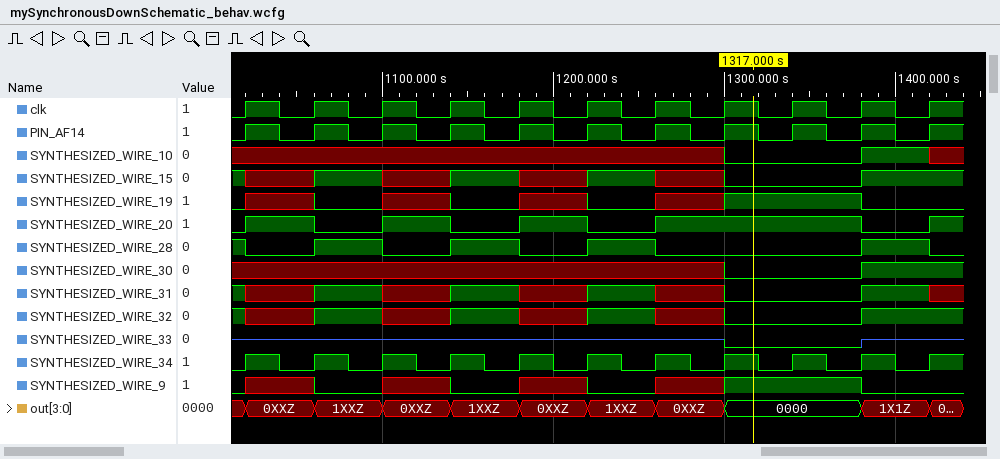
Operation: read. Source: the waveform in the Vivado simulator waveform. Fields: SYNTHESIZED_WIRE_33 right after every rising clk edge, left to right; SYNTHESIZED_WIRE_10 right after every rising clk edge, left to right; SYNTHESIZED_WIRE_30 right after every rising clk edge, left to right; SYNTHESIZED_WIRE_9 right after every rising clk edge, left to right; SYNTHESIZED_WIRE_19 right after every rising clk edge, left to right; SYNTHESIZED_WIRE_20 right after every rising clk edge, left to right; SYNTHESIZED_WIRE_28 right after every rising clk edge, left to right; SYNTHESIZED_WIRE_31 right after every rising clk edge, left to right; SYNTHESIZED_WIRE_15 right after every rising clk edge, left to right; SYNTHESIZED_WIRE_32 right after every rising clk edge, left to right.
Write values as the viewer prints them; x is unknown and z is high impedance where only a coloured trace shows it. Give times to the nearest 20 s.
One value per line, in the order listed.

z z z z z z z 0 0 z z
x x x x x x x 0 0 1 x
x x x x x x x 0 0 1 1
x 0 x 0 x 0 x 1 1 0 0
x 0 x 0 x 0 x 1 1 0 0
1 0 1 0 1 0 1 1 1 0 1
0 1 0 1 0 1 0 0 0 1 0
x 1 x 1 x 1 x 0 0 1 x
x 1 x 1 x 1 x 0 0 1 1
x 1 x 1 x 1 x 0 0 1 1
